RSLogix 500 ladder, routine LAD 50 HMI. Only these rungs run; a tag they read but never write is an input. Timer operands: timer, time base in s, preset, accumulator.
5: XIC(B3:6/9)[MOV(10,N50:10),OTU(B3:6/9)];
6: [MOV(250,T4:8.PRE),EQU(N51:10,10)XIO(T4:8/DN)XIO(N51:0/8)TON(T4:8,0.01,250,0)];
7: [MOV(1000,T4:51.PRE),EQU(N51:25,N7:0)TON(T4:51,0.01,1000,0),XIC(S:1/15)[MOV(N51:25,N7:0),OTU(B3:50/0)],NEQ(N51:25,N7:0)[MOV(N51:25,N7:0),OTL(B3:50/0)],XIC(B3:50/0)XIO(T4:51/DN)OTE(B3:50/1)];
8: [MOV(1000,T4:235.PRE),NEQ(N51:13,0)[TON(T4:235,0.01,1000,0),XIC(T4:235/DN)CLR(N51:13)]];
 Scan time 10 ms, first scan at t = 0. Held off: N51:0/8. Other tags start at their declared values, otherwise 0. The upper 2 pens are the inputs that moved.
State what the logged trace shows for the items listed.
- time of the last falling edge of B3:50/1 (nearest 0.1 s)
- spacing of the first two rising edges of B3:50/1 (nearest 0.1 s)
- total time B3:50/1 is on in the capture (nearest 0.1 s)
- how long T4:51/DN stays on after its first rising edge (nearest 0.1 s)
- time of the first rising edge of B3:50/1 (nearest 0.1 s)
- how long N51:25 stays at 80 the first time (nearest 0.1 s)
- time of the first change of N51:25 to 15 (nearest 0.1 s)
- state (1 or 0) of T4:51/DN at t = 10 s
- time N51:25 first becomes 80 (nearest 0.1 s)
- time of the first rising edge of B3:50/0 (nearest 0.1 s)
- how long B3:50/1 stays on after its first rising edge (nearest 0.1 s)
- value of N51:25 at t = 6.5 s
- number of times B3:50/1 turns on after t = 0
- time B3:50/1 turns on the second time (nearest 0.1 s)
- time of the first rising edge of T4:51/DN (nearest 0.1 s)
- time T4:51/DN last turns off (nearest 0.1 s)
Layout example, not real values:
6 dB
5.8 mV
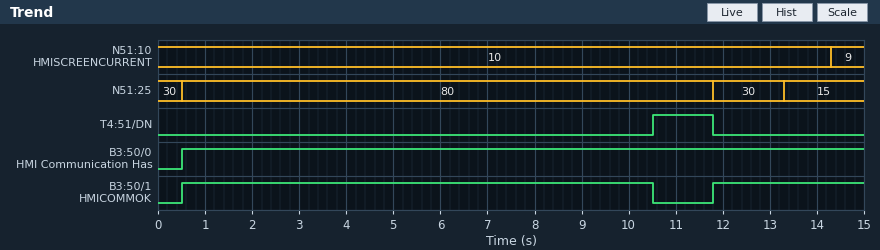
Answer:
10.5 s
11.3 s
13.2 s
1.3 s
0.5 s
11.3 s
13.3 s
0
0.5 s
0.5 s
10.0 s
80
2
11.8 s
10.5 s
11.8 s
